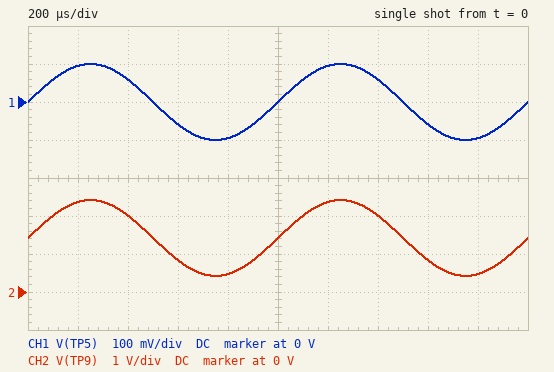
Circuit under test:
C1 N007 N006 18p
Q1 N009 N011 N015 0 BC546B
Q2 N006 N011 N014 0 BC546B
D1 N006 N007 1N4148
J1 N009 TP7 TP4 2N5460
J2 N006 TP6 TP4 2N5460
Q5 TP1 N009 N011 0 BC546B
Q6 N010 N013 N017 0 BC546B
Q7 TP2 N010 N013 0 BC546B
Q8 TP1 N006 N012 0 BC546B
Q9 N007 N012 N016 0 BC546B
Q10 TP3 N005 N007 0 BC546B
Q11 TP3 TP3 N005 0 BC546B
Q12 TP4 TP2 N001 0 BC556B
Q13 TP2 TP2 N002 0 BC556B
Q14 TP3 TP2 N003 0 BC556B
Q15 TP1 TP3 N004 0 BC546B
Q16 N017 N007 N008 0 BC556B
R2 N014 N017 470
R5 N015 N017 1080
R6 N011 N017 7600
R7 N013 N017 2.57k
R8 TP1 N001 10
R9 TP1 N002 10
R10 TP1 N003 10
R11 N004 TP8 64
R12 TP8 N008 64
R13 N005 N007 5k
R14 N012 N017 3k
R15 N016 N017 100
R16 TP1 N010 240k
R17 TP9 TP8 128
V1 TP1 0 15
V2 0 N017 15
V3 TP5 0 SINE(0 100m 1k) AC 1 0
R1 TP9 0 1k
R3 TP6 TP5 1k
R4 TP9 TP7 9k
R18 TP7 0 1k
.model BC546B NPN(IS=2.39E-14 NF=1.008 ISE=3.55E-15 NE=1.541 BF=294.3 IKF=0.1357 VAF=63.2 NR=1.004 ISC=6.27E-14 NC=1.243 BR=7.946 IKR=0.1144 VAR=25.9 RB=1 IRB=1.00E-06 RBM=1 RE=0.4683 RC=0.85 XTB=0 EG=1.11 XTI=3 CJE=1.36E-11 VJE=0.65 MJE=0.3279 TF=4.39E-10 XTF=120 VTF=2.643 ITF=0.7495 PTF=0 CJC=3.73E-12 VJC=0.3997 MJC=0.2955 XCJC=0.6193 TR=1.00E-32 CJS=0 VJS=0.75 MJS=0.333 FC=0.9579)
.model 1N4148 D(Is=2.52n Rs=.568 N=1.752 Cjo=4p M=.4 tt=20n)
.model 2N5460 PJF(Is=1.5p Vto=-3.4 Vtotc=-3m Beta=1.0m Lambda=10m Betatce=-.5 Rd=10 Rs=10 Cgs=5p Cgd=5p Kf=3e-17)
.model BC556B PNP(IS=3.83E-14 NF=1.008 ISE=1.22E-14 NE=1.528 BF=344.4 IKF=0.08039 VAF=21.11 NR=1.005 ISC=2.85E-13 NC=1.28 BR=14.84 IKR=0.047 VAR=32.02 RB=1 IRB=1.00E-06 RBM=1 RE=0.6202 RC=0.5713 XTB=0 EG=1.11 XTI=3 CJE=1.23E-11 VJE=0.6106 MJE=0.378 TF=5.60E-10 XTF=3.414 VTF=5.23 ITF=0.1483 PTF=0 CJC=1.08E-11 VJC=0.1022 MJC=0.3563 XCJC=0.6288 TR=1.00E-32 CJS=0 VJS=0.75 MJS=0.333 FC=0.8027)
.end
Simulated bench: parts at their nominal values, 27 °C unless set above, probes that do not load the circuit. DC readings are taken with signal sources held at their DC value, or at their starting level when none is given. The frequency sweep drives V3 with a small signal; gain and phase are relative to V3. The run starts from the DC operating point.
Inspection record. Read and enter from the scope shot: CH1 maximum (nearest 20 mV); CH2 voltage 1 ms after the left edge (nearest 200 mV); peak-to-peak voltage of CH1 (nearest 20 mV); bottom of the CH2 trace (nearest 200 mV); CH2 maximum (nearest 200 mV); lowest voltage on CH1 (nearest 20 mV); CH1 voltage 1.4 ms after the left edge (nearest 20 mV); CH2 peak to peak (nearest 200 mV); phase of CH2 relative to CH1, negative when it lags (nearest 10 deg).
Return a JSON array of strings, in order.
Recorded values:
["100 mV", "1.4 V", "200 mV", "400 mV", "2.4 V", "-100 mV", "60 mV", "2.0 V", "0 deg"]
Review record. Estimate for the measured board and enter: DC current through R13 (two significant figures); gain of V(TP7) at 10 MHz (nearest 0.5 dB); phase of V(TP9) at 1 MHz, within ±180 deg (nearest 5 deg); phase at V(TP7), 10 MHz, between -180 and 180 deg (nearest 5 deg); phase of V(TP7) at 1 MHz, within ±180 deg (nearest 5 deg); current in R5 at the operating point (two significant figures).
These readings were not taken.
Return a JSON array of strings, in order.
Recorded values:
["120 µA", "-14.0 dB", "-50 deg", "105 deg", "-50 deg", "130 µA"]
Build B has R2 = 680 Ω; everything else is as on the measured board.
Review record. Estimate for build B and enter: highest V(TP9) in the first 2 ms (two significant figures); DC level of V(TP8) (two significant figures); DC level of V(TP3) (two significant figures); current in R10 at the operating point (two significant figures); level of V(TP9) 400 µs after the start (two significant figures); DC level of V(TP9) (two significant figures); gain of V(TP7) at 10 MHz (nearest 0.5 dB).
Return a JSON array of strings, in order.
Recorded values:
["1.8 V", "950 mV", "1.6 V", "350 µA", "1.4 V", "830 mV", "-16.5 dB"]
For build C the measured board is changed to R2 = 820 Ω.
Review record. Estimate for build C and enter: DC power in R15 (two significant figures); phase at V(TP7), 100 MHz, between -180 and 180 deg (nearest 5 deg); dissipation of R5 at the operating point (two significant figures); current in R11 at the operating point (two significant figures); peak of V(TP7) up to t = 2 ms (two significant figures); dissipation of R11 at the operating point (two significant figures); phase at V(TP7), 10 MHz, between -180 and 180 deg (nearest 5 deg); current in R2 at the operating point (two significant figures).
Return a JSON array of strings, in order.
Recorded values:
["12 µW", "-30 deg", "31 µW", "590 µA", "150 mV", "22 µW", "100 deg", "220 µA"]
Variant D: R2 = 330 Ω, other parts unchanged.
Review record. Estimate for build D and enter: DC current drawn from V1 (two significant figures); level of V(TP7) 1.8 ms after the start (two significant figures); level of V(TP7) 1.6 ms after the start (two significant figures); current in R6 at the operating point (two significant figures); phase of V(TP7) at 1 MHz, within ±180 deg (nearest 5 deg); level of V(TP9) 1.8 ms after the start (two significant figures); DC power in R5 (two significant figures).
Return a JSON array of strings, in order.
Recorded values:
["3.5 mA", "96 mV", "130 mV", "92 µA", "-45 deg", "960 mV", "13 µW"]
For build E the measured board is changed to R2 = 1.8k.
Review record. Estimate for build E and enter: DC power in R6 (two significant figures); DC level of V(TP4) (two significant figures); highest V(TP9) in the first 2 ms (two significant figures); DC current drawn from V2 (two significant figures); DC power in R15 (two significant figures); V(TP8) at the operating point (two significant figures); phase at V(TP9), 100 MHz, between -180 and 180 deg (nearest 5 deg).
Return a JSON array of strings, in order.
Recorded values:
["97 µW", "-3.0 V", "32 mV", "2.5 mA", "14 µW", "-1.1 V", "10 deg"]
